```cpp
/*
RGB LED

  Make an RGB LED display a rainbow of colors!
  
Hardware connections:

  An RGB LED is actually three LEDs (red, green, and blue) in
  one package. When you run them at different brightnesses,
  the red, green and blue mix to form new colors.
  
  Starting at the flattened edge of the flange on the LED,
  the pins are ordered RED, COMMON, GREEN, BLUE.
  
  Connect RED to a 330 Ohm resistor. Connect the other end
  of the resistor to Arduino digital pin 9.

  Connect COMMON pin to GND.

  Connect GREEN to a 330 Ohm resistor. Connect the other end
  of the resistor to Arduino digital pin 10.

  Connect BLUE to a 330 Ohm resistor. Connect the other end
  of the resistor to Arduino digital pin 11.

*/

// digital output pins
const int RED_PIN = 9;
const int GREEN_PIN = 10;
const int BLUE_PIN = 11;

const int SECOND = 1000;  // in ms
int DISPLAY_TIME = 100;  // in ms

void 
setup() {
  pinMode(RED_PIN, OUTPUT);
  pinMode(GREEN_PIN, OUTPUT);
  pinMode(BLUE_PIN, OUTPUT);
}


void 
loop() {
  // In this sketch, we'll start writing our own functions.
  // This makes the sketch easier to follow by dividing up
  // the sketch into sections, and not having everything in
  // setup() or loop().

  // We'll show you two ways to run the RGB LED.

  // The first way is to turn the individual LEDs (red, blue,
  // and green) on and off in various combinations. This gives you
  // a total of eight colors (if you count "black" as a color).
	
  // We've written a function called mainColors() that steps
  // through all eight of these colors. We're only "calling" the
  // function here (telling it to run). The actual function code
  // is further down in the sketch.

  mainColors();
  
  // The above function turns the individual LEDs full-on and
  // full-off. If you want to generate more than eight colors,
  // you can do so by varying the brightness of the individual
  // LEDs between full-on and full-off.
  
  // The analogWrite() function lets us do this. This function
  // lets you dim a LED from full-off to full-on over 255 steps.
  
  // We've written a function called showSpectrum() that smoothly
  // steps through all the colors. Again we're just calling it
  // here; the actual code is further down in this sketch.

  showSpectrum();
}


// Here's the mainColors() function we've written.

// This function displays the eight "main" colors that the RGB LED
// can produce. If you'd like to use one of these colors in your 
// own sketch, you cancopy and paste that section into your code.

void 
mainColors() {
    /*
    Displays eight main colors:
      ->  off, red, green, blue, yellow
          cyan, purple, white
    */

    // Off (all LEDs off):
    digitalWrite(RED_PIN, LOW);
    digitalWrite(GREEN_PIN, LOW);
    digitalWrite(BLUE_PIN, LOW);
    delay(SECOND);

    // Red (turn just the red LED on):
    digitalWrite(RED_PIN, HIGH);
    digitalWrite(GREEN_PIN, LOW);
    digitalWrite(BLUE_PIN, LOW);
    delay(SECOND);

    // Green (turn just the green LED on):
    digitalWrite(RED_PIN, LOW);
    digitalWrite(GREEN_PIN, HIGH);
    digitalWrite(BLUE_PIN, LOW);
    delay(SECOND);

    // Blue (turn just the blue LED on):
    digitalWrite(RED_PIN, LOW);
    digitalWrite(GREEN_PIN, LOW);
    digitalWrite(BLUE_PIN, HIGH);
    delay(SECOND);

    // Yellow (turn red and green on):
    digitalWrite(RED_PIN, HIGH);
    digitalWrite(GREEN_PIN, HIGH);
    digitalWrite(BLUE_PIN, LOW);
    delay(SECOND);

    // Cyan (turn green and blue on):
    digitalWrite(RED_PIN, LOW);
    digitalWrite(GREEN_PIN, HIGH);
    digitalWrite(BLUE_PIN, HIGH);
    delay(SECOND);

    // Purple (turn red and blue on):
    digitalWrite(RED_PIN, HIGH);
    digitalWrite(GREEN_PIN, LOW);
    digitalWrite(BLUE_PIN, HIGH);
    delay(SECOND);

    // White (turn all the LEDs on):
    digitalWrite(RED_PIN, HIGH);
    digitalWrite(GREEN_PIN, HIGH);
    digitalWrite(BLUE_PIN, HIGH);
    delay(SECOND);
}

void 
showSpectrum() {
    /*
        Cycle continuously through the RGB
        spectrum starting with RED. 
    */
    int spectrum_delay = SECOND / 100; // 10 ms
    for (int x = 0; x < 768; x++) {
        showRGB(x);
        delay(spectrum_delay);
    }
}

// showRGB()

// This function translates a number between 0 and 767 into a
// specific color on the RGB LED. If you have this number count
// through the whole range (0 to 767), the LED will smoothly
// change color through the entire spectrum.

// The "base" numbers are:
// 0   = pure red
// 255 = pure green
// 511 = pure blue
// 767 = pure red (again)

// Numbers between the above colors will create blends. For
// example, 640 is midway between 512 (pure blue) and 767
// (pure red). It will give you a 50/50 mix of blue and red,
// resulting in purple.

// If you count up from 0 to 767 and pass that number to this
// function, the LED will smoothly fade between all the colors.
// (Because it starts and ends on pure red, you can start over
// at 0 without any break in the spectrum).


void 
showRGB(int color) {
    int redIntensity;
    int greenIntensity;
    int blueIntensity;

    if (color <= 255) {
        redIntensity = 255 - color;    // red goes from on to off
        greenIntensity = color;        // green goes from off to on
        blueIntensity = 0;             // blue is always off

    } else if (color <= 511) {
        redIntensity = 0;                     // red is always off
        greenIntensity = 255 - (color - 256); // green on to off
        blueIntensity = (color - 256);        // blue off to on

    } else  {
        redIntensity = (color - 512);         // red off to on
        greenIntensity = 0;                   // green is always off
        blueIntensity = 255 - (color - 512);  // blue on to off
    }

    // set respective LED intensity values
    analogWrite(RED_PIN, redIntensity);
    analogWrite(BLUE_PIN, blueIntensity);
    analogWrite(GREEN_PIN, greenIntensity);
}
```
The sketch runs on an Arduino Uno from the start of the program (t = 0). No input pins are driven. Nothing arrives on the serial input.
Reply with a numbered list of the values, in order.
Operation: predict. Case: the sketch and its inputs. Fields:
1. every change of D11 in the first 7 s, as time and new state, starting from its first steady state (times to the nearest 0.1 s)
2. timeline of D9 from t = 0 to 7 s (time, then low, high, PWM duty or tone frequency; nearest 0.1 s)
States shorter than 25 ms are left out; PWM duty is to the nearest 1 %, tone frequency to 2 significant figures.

1. 0 s low; 3 s high; 4 s low; 5 s high
2. 0 s low; 1 s high; 2 s low; 4 s high; 5 s low; 6 s high
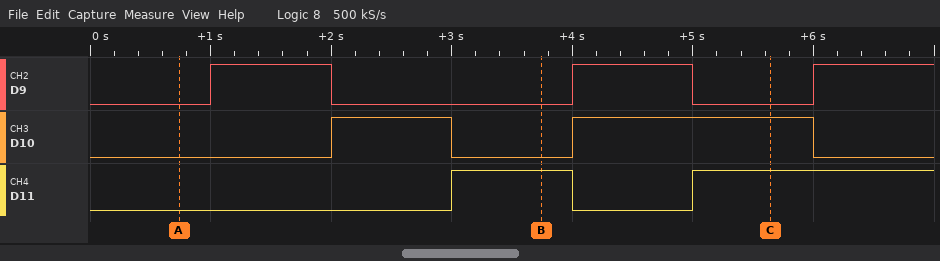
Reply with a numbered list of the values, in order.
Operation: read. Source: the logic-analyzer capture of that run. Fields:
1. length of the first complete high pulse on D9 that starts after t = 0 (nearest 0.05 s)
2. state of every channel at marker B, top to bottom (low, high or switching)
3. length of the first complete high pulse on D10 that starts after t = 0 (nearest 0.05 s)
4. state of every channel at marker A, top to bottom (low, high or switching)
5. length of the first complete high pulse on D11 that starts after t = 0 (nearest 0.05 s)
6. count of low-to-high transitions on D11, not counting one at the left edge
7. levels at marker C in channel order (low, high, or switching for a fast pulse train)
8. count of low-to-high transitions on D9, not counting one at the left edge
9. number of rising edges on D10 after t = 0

1. 1.00 s
2. D9 low, D10 low, D11 high
3. 1.00 s
4. D9 low, D10 low, D11 low
5. 1.00 s
6. 2
7. D9 low, D10 high, D11 high
8. 3
9. 2
